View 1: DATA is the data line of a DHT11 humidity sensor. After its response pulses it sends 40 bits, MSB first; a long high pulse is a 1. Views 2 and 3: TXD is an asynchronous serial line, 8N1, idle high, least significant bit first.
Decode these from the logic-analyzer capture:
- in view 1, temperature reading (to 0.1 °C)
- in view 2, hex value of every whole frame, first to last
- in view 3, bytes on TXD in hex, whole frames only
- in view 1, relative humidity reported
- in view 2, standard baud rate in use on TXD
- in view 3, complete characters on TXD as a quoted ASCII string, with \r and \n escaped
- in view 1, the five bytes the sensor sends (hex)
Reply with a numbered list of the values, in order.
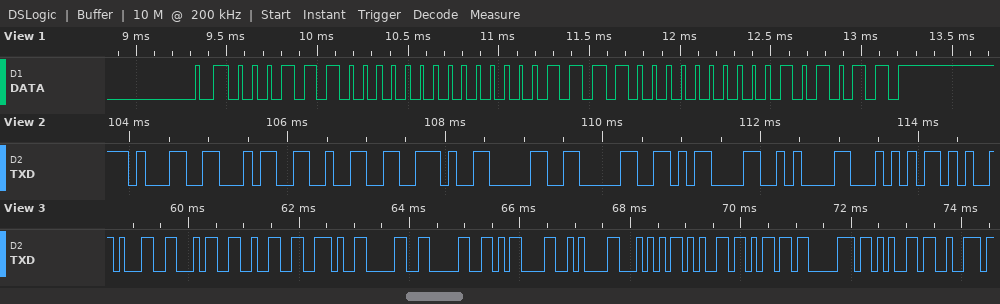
1. 15.0 °C
2. 31 34 32 2E 30 30 0D 0A 54
3. 0x31 0x34 0x32 0x2E 0x30 0x30 0x0D 0x0A 0x54 0x65 0x6D 0x70 0x65 0x72
4. 28 %
5. 9600 baud
6. "142.00\r\nTemper"
7. 1C 00 0F 00 2B
